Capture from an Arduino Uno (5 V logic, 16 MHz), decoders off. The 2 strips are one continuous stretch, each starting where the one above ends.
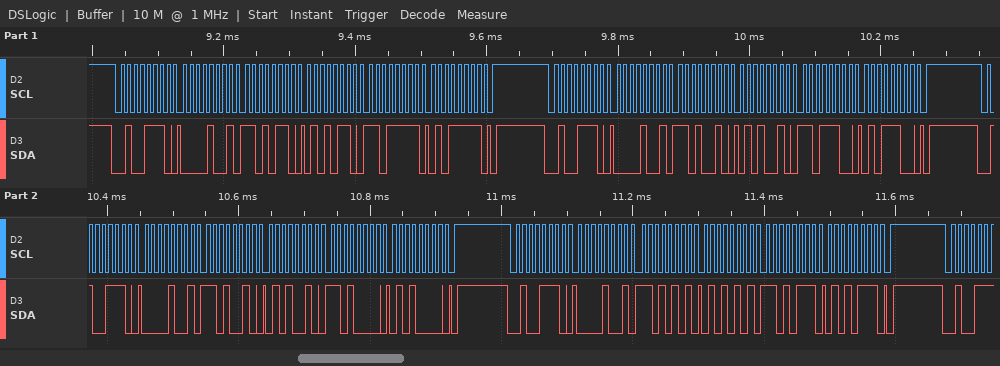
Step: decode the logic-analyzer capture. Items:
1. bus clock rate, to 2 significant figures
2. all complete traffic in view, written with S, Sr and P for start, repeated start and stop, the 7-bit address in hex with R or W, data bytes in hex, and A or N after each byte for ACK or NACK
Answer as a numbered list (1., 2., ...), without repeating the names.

1. 100 kHz
2. S 27W A 09 A D6 A 56 A DF A 5F A P S 27W A 09 A D2 A 52 A DC A 5C A P S 27W A 09 A D2 A 52 A D0 A 50 A P S 27W A 09 A D5 A 55 A D7 A 57 A P
